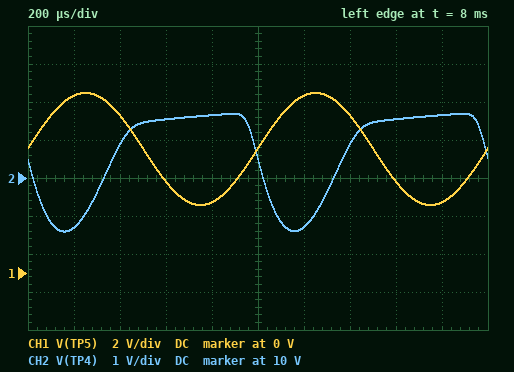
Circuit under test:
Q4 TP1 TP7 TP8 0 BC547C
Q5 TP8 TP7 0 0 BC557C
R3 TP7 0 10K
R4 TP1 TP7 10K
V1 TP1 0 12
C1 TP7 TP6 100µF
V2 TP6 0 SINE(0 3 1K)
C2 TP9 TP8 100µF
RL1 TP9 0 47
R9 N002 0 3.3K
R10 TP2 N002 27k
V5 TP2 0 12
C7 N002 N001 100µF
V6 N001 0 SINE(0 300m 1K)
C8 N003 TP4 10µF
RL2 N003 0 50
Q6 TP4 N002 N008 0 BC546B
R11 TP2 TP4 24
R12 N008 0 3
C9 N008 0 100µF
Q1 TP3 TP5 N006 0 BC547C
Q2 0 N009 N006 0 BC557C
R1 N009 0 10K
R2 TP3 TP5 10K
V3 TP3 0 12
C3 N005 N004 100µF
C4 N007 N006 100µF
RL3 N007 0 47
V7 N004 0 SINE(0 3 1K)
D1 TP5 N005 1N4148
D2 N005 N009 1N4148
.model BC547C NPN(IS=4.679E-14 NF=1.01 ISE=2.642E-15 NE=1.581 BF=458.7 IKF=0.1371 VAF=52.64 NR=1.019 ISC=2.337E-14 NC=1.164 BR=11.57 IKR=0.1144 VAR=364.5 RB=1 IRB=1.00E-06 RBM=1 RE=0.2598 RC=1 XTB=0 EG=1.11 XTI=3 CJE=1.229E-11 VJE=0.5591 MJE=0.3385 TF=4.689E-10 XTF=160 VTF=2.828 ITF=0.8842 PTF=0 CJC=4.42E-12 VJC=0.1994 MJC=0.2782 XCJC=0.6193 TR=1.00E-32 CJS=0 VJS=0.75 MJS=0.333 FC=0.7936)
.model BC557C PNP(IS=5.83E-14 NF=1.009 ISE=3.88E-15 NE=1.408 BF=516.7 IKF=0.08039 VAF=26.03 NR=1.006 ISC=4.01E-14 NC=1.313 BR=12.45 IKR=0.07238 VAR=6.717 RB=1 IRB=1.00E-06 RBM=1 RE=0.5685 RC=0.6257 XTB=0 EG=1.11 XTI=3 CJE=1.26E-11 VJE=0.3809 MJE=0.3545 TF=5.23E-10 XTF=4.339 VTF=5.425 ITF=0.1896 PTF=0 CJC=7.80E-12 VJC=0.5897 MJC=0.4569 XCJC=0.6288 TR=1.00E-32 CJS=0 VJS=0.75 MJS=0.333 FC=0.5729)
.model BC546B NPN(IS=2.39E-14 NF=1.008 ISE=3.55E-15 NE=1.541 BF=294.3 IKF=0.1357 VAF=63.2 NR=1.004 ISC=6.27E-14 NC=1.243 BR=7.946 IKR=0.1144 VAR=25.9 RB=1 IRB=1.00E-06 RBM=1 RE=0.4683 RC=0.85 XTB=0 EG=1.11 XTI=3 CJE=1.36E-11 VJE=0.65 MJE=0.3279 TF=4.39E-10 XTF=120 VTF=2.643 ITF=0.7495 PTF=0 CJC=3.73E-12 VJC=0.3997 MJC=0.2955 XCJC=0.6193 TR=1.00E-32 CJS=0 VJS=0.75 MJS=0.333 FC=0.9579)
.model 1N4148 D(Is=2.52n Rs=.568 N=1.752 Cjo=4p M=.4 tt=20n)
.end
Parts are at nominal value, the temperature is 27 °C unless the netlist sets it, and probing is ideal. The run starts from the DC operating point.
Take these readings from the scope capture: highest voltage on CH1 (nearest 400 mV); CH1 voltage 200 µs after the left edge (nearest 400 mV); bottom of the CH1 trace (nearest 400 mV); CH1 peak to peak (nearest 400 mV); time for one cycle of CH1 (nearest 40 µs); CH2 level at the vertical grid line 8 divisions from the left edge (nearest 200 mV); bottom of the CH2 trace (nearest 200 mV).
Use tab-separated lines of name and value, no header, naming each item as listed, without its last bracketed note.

highest voltage on CH1	9.6 V
CH1 voltage 200 µs after the left edge	9.2 V
bottom of the CH1 trace	3.6 V
CH1 peak to peak	6.0 V
time for one cycle of CH1	1.00 ms
CH2 level at the vertical grid line 8 divisions from the left edge	11.6 V
bottom of the CH2 trace	8.6 V
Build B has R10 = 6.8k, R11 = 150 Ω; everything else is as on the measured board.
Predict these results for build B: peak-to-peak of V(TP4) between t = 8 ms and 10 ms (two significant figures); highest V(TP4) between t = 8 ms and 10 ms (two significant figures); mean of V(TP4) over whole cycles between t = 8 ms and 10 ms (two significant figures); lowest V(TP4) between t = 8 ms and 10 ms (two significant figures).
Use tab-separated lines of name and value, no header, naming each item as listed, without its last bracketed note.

peak-to-peak of V(TP4) between t = 8 ms and 10 ms	6.4 V
highest V(TP4) between t = 8 ms and 10 ms	6.9 V
mean of V(TP4) over whole cycles between t = 8 ms and 10 ms	4.3 V
lowest V(TP4) between t = 8 ms and 10 ms	460 mV
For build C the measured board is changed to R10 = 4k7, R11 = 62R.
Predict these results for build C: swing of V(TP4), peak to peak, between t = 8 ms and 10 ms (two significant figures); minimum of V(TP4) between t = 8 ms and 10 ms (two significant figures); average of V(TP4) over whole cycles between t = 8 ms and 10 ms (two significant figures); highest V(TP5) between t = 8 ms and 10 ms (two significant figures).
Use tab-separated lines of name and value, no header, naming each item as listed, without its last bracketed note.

swing of V(TP4), peak to peak, between t = 8 ms and 10 ms	7.4 V
minimum of V(TP4) between t = 8 ms and 10 ms	850 mV
average of V(TP4) over whole cycles between t = 8 ms and 10 ms	4.7 V
highest V(TP5) between t = 8 ms and 10 ms	9.5 V
